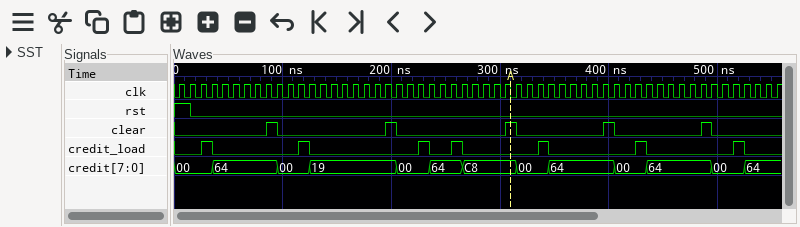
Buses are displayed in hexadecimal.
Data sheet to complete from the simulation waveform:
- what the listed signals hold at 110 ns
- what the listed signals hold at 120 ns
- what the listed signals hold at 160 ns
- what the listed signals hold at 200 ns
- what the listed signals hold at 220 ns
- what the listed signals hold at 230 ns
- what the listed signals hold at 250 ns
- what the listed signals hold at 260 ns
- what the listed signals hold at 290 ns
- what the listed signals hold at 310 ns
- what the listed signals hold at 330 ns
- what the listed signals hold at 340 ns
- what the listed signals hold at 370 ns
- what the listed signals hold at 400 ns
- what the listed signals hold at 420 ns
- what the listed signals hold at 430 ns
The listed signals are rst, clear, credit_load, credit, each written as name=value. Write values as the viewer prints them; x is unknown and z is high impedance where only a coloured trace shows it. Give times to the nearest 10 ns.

rst=0, clear=0, credit_load=0, credit=00
rst=0, clear=0, credit_load=1, credit=00
rst=0, clear=0, credit_load=0, credit=19
rst=0, clear=1, credit_load=0, credit=19
rst=0, clear=0, credit_load=0, credit=00
rst=0, clear=0, credit_load=1, credit=00
rst=0, clear=0, credit_load=0, credit=64
rst=0, clear=0, credit_load=1, credit=64
rst=0, clear=0, credit_load=0, credit=C8
rst=0, clear=1, credit_load=0, credit=C8
rst=0, clear=0, credit_load=0, credit=00
rst=0, clear=0, credit_load=1, credit=00
rst=0, clear=0, credit_load=0, credit=64
rst=0, clear=1, credit_load=0, credit=64
rst=0, clear=0, credit_load=0, credit=00
rst=0, clear=0, credit_load=1, credit=00
